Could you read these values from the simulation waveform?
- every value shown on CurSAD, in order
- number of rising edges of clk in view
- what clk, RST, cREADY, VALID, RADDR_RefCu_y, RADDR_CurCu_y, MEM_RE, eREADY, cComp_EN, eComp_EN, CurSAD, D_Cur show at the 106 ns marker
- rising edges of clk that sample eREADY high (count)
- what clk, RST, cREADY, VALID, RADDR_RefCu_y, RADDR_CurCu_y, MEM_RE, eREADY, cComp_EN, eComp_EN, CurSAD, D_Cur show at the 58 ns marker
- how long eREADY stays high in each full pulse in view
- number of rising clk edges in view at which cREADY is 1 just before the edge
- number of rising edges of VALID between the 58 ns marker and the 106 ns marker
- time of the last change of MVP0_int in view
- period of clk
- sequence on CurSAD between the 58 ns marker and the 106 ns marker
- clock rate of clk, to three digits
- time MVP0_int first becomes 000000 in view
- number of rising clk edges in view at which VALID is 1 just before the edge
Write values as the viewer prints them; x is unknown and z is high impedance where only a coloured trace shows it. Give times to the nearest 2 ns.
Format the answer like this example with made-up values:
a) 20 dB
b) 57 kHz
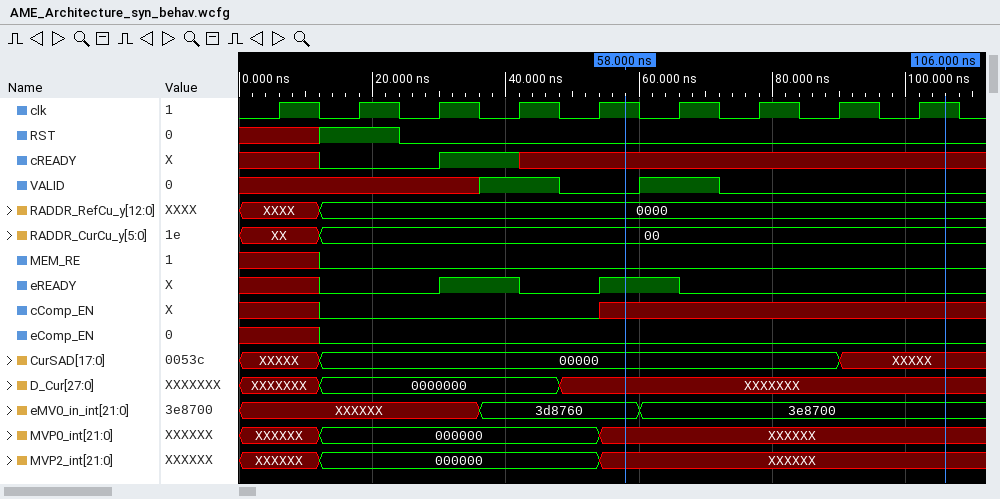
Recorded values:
a) XXXXX, 00000, XXXXX
b) 9
c) clk=1, RST=0, cREADY=x, VALID=0, RADDR_RefCu_y=0000, RADDR_CurCu_y=00, MEM_RE=0, eREADY=0, cComp_EN=x, eComp_EN=0, CurSAD=XXXXX, D_Cur=XXXXXXX
d) 2
e) clk=1, RST=0, cREADY=x, VALID=0, RADDR_RefCu_y=0000, RADDR_CurCu_y=00, MEM_RE=0, eREADY=1, cComp_EN=x, eComp_EN=0, CurSAD=00000, D_Cur=XXXXXXX
f) 12 ns, 12 ns
g) 1
h) 1
i) 54 ns
j) 12 ns
k) 00000, XXXXX
l) 83.3 MHz
m) 12 ns
n) 2
